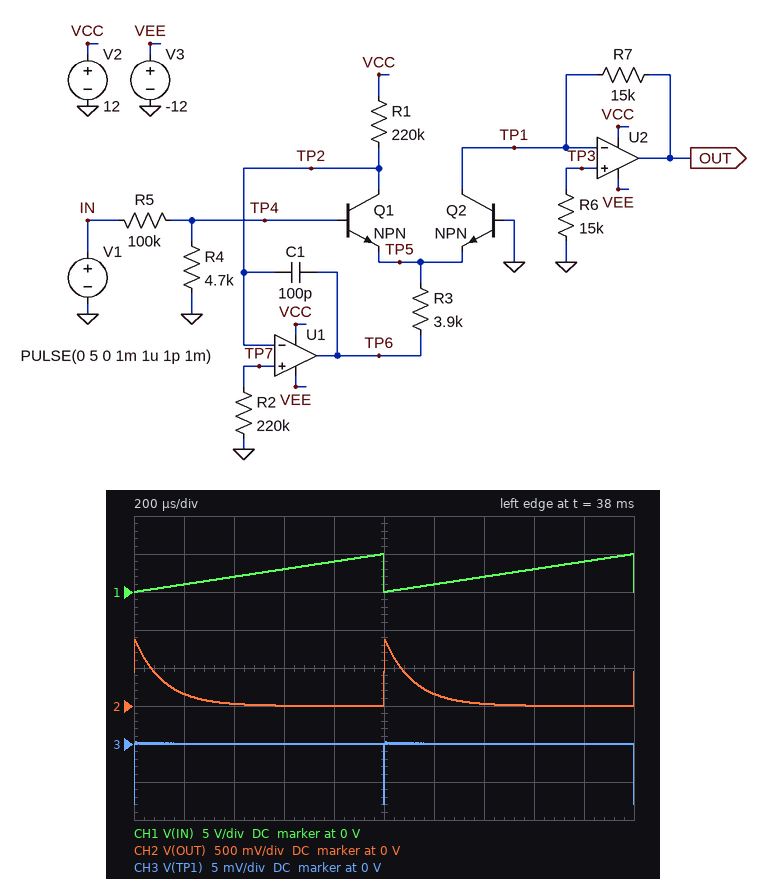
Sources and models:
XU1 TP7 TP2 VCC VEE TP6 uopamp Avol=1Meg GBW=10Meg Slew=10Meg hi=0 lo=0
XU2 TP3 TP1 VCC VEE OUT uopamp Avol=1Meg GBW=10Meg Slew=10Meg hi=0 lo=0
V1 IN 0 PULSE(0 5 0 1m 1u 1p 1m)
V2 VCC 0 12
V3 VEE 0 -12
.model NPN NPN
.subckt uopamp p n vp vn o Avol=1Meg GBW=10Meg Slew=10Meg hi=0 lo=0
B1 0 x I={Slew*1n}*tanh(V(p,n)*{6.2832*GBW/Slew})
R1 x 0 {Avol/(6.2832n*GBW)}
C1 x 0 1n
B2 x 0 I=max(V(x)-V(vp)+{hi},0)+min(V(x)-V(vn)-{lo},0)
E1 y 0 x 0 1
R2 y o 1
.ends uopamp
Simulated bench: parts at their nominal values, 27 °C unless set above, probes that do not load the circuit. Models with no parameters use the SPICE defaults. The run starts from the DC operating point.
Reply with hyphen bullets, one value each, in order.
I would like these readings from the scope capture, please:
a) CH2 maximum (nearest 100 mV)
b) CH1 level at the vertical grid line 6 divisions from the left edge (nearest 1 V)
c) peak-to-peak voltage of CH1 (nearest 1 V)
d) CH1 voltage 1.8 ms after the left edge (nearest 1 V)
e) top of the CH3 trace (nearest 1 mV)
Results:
- 900 mV
- 1 V
- 5 V
- 4 V
- 0 V
